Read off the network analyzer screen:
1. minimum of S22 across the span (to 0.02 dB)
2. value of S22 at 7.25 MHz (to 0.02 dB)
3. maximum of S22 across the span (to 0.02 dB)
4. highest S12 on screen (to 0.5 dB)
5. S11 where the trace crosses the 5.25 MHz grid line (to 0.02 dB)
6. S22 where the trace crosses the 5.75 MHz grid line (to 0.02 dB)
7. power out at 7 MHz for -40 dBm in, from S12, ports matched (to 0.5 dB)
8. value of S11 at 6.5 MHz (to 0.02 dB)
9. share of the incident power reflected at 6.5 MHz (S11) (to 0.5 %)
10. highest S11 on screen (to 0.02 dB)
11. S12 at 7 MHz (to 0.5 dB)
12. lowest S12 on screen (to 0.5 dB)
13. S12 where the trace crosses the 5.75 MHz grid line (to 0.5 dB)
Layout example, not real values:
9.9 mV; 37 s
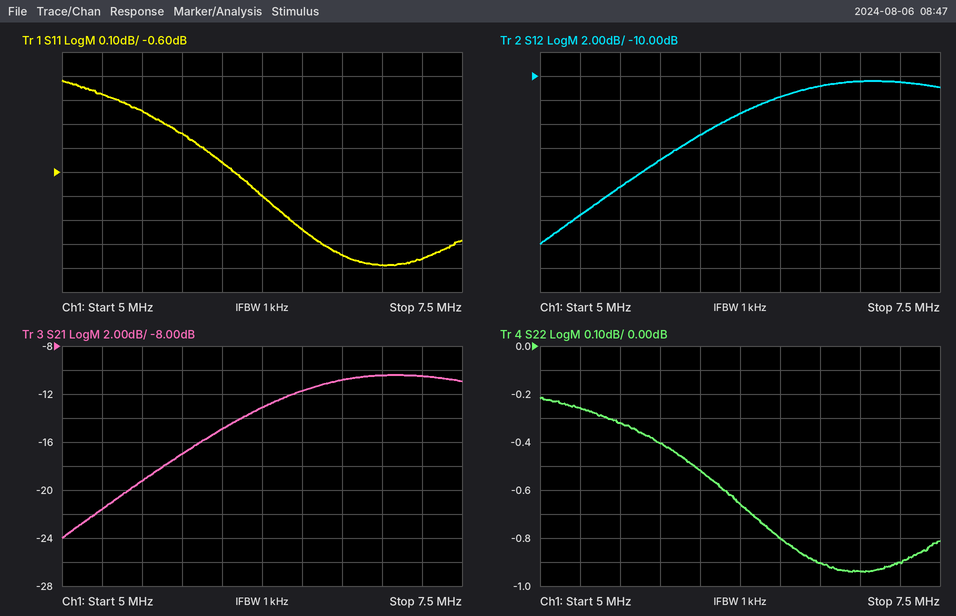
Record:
-0.94 dB; -0.90 dB; -0.22 dB; -10.5 dB; -0.28 dB; -0.40 dB; -50.5 dBm; -0.84 dB; 82.5 %; -0.22 dB; -10.5 dB; -24.0 dB; -17.0 dB
